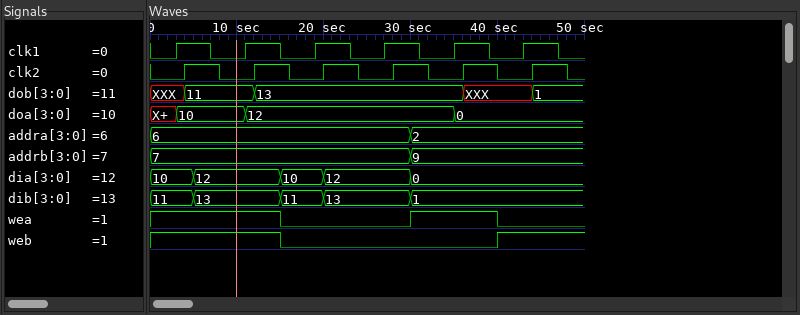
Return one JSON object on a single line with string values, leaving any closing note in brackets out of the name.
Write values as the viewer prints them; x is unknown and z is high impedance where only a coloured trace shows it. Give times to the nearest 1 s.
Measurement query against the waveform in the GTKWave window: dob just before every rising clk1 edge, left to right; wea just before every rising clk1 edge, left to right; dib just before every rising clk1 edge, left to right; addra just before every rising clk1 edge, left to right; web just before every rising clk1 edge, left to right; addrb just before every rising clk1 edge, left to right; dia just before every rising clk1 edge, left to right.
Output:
{"dob just before every rising clk1 edge, left to right": "XXX, 11, 13, 13, 13, XXX", "wea just before every rising clk1 edge, left to right": "1 1 0 0 1 0", "dib just before every rising clk1 edge, left to right": "11, 13, 11, 13, 1, 1", "addra just before every rising clk1 edge, left to right": "6, 6, 6, 6, 2, 2", "web just before every rising clk1 edge, left to right": "1 1 0 0 0 1", "addrb just before every rising clk1 edge, left to right": "7, 7, 7, 7, 9, 9", "dia just before every rising clk1 edge, left to right": "10, 12, 10, 12, 0, 0"}
